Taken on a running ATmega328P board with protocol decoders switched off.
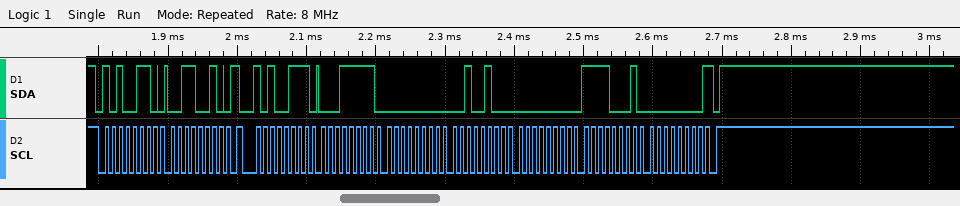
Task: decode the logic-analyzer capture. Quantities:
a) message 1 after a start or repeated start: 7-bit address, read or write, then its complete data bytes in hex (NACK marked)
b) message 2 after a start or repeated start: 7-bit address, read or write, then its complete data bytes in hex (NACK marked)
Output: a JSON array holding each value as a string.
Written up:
["0x53 write: 32", "0x53 read: 1F 00 24 00 F1 00 NACK"]
